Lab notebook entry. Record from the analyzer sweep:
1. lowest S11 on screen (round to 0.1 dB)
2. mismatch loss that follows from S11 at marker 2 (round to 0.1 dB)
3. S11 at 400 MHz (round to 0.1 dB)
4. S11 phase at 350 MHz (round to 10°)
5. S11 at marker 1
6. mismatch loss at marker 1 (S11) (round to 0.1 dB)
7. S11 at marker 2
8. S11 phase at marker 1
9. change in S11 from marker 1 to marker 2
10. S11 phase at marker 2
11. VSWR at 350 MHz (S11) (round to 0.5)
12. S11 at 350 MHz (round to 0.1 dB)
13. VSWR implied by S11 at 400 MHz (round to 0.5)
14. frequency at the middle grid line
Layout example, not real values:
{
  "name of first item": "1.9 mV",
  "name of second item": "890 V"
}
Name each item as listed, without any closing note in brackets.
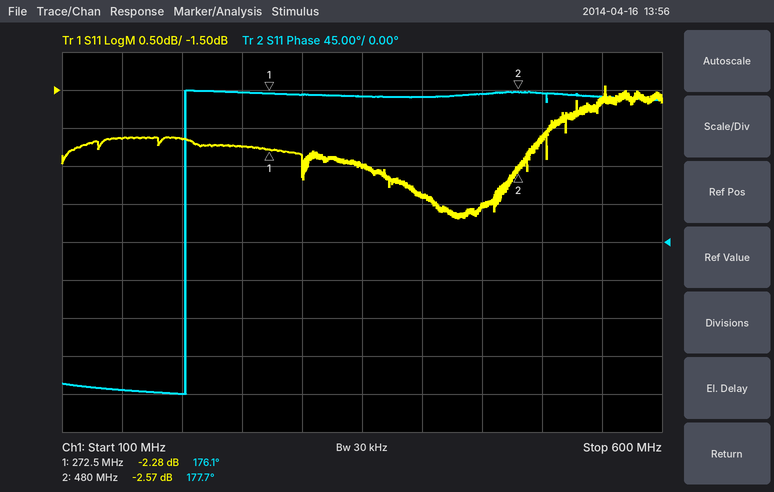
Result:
{
  "lowest S11 on screen": "-3.2 dB",
  "mismatch loss that follows from S11 at marker 2": "3.5 dB",
  "S11 at 400 MHz": "-2.9 dB",
  "S11 phase at 350 MHz": "170°",
  "S11 at marker 1": "-2.28 dB",
  "mismatch loss at marker 1 (S11)": "3.9 dB",
  "S11 at marker 2": "-2.57 dB",
  "S11 phase at marker 1": "176.1°",
  "change in S11 from marker 1 to marker 2": "-0.29 dB",
  "S11 phase at marker 2": "177.7°",
  "VSWR at 350 MHz (S11)": "7.0",
  "S11 at 350 MHz": "-2.5 dB",
  "VSWR implied by S11 at 400 MHz": "6.0",
  "frequency at the middle grid line": "350 MHz"
}
